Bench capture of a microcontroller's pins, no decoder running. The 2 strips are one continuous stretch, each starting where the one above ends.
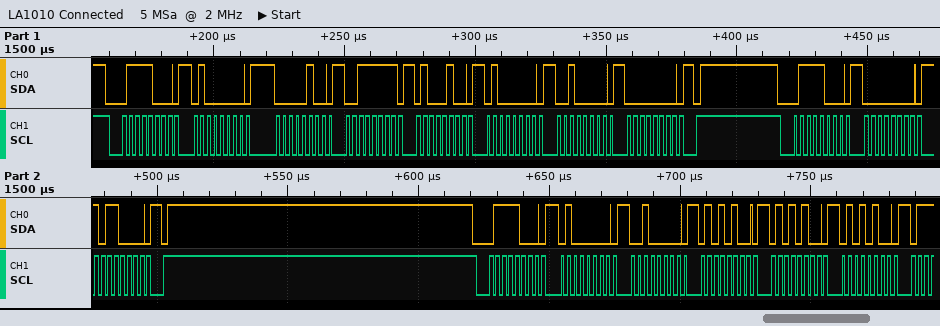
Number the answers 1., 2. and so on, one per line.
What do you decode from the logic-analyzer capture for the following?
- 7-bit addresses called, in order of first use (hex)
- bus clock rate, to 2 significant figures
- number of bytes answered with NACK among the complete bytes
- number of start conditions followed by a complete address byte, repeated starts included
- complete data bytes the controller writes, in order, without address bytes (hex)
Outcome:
1. 0x3C
2. 400 kHz
3. 0
4. 3
5. 40 04 3F 44 40 20 00 00 B0 40 20 54 54 54
